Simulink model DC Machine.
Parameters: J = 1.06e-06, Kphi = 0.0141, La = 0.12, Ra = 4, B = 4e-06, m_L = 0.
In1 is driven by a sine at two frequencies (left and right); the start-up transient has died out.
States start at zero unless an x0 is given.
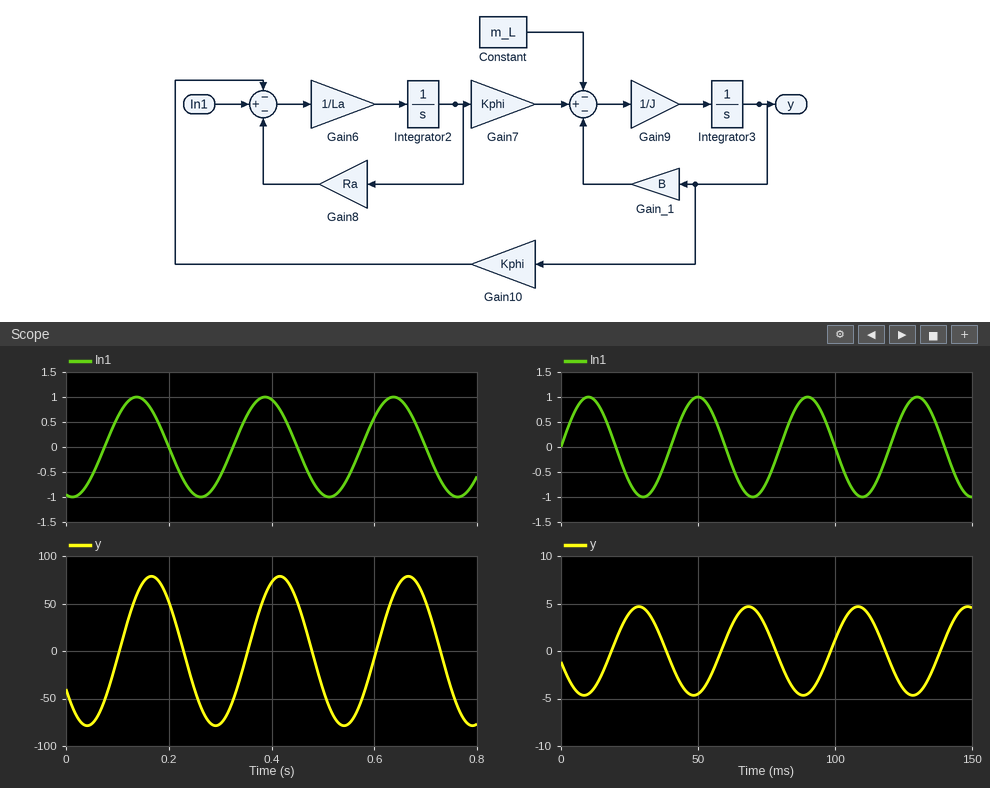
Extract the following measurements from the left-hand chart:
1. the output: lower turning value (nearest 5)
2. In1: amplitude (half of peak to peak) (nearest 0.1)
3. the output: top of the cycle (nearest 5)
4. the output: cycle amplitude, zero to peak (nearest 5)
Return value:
-80
1.0
80
80
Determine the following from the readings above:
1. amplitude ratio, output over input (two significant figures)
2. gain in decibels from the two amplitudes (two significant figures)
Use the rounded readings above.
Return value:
80
38 dB
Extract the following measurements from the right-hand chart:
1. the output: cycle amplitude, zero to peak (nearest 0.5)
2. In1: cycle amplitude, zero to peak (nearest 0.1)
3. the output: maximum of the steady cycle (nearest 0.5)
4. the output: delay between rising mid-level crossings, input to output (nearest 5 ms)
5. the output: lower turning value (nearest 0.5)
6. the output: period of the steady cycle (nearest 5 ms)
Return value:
4.5
1.0
4.5
20 ms
-4.5
40 ms
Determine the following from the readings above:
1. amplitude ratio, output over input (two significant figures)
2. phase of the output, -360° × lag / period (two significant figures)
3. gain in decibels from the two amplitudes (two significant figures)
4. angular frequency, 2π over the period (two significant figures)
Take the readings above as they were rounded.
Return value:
4.5
-180°
13 dB
0.16 rad/ms
